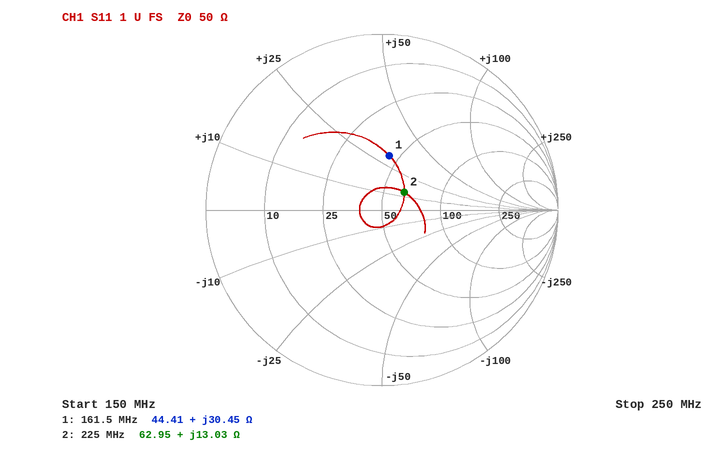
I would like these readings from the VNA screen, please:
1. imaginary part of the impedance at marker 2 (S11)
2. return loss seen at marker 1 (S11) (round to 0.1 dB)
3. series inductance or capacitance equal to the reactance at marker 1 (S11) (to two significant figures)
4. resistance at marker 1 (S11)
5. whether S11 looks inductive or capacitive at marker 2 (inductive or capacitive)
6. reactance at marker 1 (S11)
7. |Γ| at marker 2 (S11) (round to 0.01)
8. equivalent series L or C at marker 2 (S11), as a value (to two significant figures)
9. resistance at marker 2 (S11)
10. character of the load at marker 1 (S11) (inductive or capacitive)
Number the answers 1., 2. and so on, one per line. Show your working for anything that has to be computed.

1. +13.03 Ω
2. 10.1 dB
3. L = 30.45 Ω/(2π × 161.5 MHz) ≈ 30 nH
4. 44.41 Ω
5. inductive
6. +30.45 Ω
7. 0.16
8. L = 13.03 Ω/(2π × 225 MHz) ≈ 9.2 nH
9. 62.95 Ω
10. inductive
